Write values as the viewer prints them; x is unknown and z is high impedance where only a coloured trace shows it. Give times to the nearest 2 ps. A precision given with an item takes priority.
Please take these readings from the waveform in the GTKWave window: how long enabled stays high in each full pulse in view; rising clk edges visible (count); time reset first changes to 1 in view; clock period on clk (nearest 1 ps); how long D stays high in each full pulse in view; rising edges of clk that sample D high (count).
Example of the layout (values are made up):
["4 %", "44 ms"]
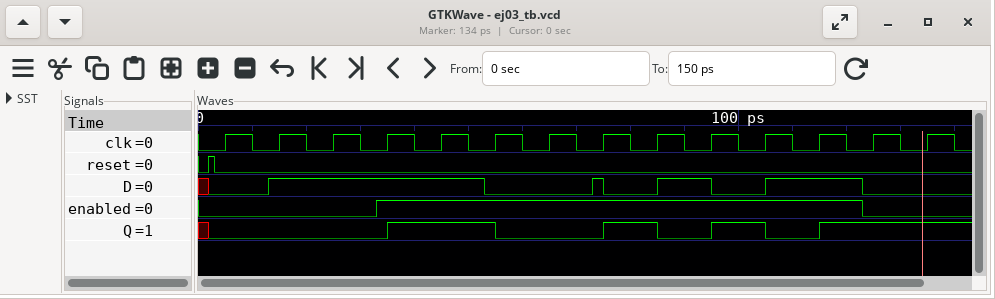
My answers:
["90 ps", "14", "2 ps", "10 ps", "40 ps, 2 ps, 10 ps, 18 ps", "7"]
